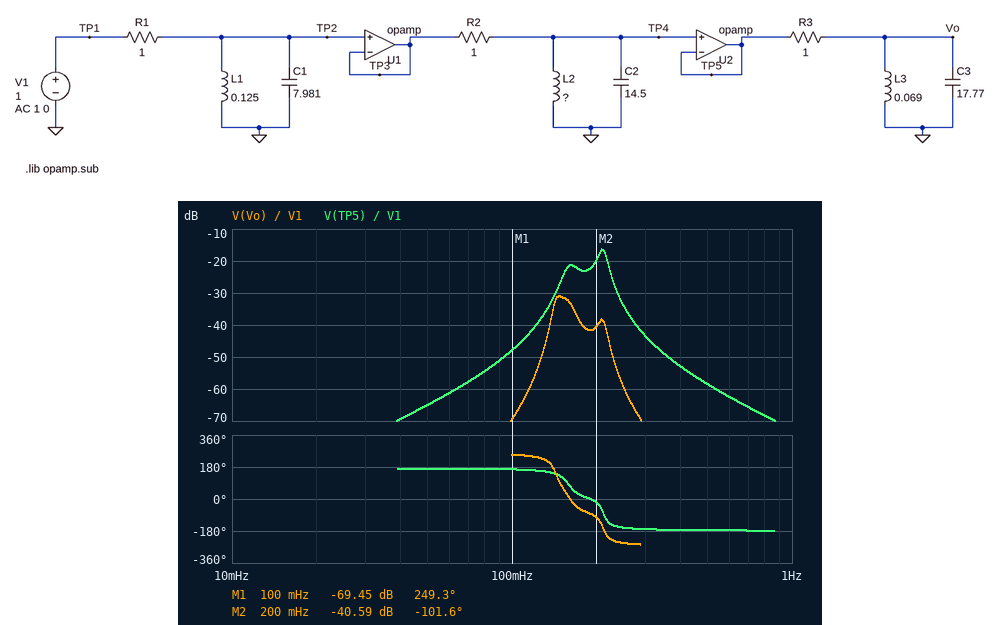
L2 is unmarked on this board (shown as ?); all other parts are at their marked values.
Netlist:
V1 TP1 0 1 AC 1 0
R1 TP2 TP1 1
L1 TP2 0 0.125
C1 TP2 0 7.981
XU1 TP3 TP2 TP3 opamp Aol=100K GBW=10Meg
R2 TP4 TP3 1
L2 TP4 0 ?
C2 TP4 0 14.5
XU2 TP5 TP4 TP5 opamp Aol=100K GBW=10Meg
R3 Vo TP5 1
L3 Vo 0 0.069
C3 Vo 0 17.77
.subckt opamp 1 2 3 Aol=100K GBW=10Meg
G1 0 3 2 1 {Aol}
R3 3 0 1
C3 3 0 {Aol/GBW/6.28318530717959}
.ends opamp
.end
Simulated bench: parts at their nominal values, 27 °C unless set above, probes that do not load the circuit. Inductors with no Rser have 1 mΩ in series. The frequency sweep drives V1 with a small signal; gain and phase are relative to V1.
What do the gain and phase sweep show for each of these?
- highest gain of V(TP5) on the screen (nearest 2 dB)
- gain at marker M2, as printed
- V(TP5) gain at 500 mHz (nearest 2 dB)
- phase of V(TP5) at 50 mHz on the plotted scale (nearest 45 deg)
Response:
-16 dB
-40.59 dB
-58 dB
180 deg
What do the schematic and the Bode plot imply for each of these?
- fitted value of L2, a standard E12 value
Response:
39 mH
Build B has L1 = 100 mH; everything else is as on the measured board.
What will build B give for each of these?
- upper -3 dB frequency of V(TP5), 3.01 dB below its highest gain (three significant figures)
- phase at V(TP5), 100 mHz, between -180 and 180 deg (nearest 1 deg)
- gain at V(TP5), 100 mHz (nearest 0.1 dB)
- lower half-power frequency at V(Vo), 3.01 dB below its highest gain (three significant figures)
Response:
217 mHz
169 deg
-50.8 dB
167 mHz
